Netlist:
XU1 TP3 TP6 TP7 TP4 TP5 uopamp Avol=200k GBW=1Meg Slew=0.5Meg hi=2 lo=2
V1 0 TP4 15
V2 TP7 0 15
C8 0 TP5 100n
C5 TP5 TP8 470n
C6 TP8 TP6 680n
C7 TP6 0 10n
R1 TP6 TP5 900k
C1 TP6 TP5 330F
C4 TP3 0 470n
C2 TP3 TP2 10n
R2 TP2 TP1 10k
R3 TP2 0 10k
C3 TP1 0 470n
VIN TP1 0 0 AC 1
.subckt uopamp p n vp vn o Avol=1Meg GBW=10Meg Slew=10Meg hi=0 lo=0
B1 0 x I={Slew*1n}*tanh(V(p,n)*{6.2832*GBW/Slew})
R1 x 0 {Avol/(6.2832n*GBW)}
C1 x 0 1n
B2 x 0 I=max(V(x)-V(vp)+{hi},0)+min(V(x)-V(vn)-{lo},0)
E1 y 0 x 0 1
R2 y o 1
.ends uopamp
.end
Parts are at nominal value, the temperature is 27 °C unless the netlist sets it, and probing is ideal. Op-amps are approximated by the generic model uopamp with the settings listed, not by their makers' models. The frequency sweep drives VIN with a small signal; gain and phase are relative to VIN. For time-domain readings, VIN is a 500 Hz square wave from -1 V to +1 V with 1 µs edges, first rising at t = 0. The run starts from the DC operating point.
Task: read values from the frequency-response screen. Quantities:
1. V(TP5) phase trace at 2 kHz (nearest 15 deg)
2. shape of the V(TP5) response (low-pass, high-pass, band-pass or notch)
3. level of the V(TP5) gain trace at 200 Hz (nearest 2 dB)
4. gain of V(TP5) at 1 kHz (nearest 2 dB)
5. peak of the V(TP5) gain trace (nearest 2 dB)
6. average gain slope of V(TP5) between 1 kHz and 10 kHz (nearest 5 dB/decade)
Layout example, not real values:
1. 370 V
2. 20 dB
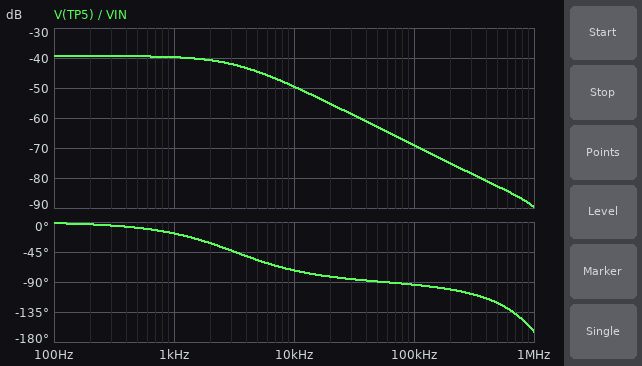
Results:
1. -30 deg
2. low-pass
3. -40 dB
4. -40 dB
5. -40 dB
6. -10 dB/decade
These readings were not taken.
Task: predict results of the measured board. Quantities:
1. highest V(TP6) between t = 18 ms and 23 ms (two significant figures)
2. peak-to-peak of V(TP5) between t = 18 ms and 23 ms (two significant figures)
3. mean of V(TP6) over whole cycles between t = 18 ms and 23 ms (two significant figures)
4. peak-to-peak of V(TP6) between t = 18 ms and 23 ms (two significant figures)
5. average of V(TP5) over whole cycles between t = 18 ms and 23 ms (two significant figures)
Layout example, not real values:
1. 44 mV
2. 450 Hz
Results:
1. 21 mV
2. 22 mV
3. 10 mV
4. 21 mV
5. 11 mV
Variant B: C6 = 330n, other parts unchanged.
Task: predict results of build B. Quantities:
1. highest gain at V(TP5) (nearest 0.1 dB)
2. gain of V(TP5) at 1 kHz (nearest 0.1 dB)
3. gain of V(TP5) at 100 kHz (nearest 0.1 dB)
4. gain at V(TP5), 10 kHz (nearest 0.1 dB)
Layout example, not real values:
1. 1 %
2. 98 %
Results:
1. -39.2 dB
2. -39.6 dB
3. -69.0 dB
4. -49.4 dB
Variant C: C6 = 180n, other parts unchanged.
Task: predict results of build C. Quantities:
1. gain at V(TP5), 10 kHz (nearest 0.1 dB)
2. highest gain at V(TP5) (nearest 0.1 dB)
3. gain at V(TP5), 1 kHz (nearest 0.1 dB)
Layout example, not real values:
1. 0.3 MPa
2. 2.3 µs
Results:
1. -49.2 dB
2. -39.0 dB
3. -39.4 dB
